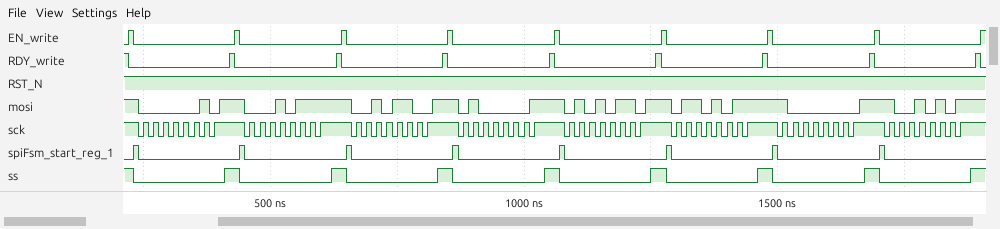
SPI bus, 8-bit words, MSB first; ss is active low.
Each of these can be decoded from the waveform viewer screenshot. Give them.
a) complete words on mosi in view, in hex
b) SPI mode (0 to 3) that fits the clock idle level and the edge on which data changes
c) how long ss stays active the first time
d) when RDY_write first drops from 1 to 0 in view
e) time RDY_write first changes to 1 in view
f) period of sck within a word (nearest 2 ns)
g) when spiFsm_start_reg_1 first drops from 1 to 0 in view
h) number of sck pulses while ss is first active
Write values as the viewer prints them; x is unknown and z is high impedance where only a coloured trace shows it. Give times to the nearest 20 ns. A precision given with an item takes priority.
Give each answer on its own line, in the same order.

02, 17, 2C, 41, 56, 6B, 80, 95
3
180 ns
220 ns
420 ns
20 ns
240 ns
8
